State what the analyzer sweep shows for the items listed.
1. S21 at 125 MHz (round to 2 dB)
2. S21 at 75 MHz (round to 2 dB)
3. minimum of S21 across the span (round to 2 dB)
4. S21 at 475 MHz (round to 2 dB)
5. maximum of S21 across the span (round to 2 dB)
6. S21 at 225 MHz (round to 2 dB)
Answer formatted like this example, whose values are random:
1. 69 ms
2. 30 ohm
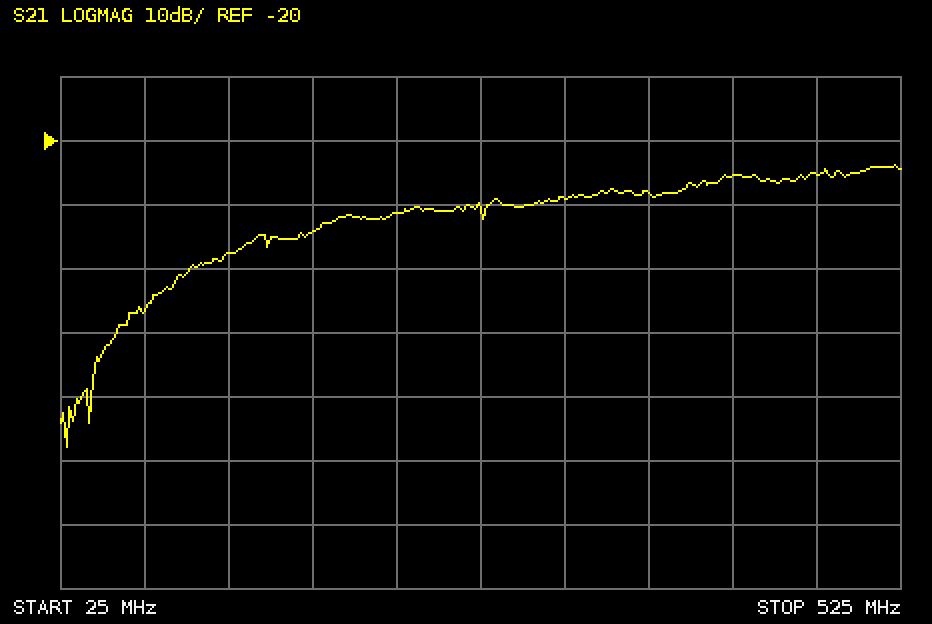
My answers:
1. -38 dB
2. -46 dB
3. -68 dB
4. -26 dB
5. -24 dB
6. -32 dB
